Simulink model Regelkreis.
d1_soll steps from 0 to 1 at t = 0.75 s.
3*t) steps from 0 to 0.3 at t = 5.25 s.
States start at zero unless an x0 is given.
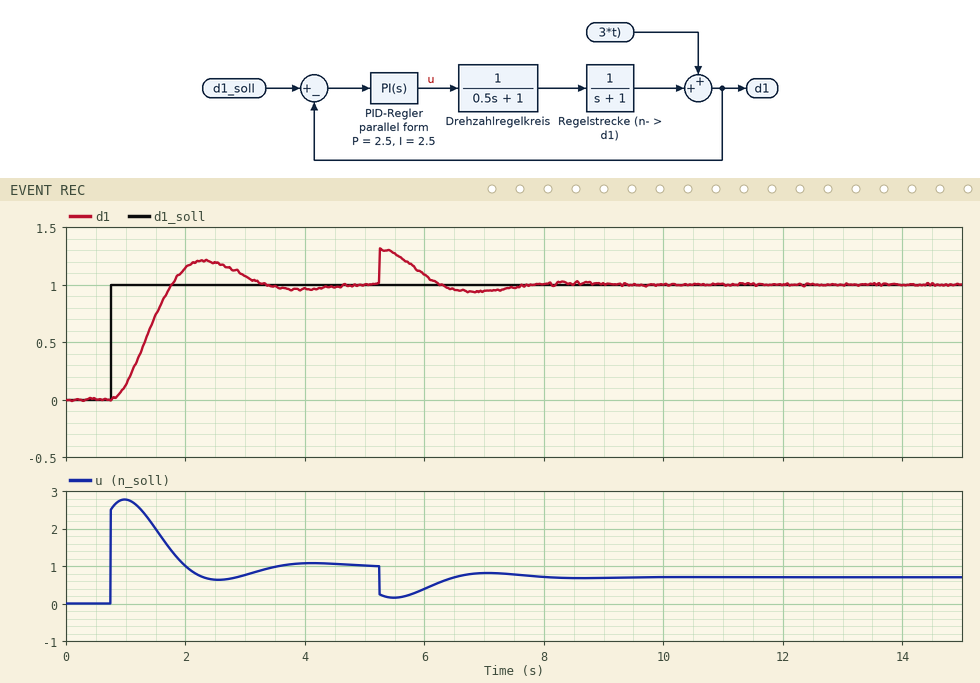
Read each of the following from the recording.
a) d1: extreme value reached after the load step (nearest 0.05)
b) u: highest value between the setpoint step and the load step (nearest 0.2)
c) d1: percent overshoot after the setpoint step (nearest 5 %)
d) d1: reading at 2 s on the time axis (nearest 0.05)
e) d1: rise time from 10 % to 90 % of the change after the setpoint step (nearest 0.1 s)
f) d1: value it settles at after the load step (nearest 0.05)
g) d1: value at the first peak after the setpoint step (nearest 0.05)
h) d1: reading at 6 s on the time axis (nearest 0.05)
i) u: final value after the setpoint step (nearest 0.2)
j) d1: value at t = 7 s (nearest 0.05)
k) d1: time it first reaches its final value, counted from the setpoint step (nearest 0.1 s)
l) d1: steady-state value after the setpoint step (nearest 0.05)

1.30
2.8
20 %
1.15
0.7 s
1.00
1.20
1.10
1.0
0.95
1.0 s
1.00
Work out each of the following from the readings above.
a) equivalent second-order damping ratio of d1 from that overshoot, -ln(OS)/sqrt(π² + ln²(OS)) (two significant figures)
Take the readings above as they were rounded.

0.46
